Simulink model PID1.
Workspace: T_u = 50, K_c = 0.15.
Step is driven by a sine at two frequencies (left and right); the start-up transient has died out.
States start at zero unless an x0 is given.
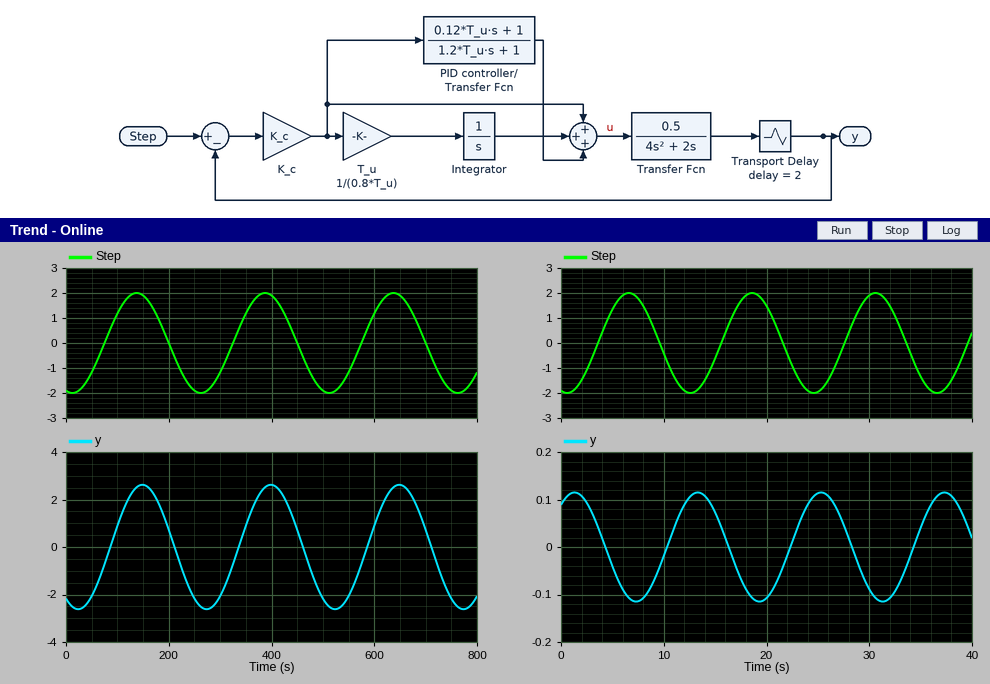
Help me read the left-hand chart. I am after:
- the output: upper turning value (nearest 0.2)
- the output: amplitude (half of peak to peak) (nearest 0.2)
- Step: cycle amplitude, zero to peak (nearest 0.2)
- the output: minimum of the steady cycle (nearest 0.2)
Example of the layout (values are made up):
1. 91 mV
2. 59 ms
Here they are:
1. 2.6
2. 2.6
3. 2.0
4. -2.6
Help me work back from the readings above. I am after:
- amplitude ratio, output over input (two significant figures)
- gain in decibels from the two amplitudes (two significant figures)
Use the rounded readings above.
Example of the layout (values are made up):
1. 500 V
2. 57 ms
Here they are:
1. 1.3
2. 2.3 dB
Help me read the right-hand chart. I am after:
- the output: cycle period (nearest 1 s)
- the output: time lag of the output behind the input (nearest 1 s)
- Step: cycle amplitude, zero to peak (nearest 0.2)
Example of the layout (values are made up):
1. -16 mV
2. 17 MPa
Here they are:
1. 12 s
2. 7 s
3. 2.0
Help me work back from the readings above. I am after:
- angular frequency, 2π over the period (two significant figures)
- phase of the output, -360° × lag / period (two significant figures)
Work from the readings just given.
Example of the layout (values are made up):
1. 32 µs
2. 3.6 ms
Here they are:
1. 0.52 rad/s
2. -210°
